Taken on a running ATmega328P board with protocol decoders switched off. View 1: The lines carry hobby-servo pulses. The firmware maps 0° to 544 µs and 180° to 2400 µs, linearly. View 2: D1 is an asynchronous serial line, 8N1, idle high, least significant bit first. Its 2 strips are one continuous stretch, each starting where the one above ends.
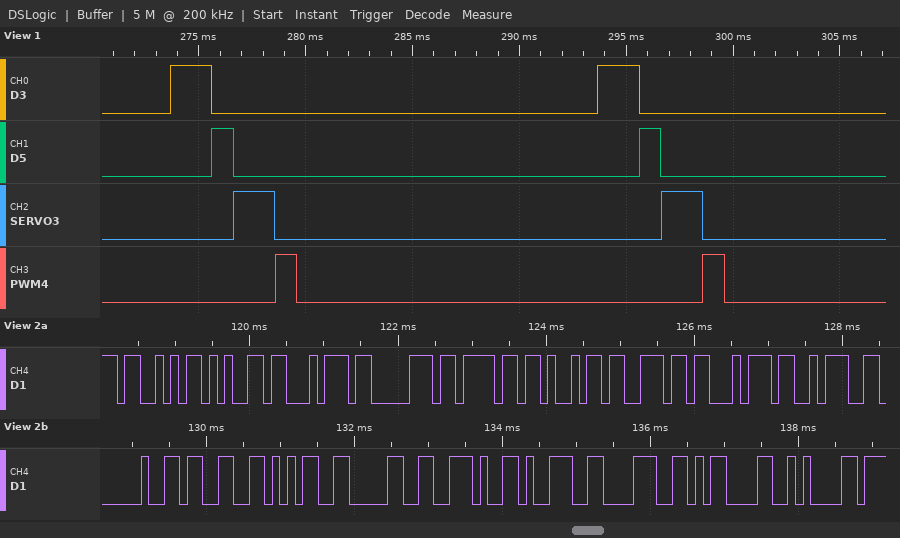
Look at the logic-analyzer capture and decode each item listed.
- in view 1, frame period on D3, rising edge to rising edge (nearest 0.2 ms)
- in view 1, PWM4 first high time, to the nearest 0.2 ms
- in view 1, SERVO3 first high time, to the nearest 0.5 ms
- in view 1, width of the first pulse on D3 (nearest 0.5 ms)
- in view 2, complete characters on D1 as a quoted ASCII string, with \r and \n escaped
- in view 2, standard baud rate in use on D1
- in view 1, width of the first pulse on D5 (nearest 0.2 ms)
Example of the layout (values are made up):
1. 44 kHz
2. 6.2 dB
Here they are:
1. 20.0 ms
2. 1.0 ms
3. 2.0 ms
4. 2.0 ms
5. "Setpoint: 350.98\r\n"
6. 9600 baud
7. 1.0 ms
